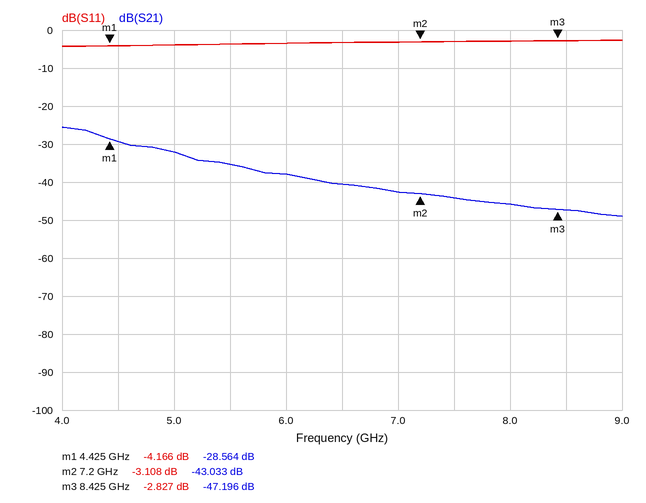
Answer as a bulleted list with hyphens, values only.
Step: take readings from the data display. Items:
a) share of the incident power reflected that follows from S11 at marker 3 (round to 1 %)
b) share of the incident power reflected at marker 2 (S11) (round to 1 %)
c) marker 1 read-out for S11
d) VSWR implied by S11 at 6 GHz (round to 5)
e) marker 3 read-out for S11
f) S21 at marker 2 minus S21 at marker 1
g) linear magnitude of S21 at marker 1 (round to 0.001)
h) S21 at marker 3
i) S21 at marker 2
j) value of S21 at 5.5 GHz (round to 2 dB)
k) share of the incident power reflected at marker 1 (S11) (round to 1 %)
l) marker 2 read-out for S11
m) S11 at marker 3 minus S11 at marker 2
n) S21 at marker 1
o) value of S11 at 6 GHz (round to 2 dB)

- 52 %
- 49 %
- -4.166 dB
- 5
- -2.827 dB
- -14.469 dB
- 0.037
- -47.196 dB
- -43.033 dB
- -36 dB
- 38 %
- -3.108 dB
- 0.281 dB
- -28.564 dB
- -4 dB
